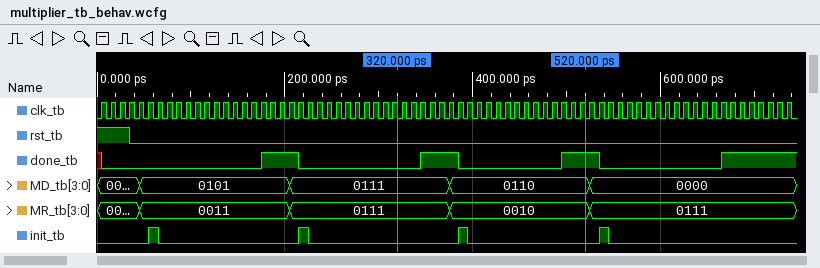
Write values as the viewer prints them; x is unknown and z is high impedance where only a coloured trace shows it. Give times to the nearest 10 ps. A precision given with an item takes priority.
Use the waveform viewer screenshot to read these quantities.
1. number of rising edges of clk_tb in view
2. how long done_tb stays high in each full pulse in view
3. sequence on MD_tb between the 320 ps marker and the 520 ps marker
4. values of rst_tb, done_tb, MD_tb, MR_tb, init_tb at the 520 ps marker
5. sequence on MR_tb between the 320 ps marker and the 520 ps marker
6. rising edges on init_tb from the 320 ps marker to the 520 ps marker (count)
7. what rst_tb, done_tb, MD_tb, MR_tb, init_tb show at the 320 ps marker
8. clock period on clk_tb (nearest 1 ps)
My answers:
74
40 ps, 40 ps, 40 ps
0111, 0110
rst_tb=0, done_tb=1, MD_tb=0110, MR_tb=0010, init_tb=0
0111, 0010
1
rst_tb=0, done_tb=0, MD_tb=0111, MR_tb=0111, init_tb=0
10 ps
